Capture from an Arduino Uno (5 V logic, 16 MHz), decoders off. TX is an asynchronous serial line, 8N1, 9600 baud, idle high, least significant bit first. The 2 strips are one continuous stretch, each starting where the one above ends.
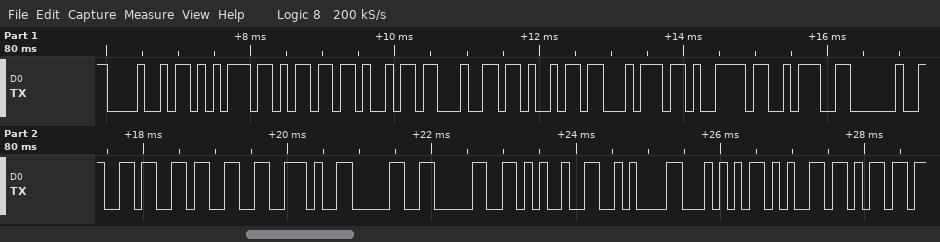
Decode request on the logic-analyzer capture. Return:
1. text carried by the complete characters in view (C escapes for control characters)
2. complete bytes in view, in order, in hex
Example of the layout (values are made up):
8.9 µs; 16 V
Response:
"Humidity: 63.00%\nTem"; 48 75 6D 69 64 69 74 79 3A 20 36 33 2E 30 30 25 0A 54 65 6D
